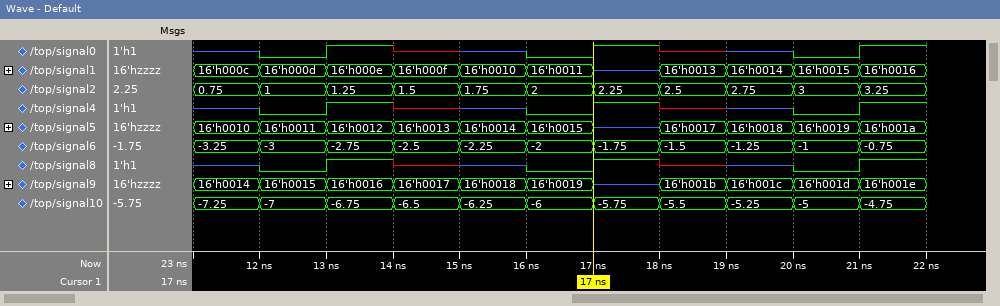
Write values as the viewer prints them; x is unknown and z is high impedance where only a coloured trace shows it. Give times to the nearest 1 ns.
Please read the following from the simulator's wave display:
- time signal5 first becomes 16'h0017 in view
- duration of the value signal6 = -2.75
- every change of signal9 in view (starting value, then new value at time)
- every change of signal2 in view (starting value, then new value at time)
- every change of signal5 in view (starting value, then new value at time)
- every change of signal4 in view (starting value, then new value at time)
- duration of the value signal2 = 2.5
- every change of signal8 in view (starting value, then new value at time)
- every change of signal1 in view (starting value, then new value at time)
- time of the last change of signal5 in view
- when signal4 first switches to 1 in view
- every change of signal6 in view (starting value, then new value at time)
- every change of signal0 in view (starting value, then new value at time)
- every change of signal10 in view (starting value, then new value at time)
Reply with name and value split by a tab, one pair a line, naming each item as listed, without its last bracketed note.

time signal5 first becomes 16'h0017 in view	18 ns
duration of the value signal6 = -2.75	1 ns
every change of signal9 in view	16'h0014, 16'h0015 at 12 ns, 16'h0016 at 13 ns, 16'h0017 at 14 ns, 16'h0018 at 15 ns, 16'h0019 at 16 ns, z at 17 ns, 16'h001b at 18 ns, 16'h001c at 19 ns, 16'h001d at 20 ns, 16'h001e at 21 ns
every change of signal2 in view	0.75, 1 at 12 ns, 1.25 at 13 ns, 1.5 at 14 ns, 1.75 at 15 ns, 2 at 16 ns, 2.25 at 17 ns, 2.5 at 18 ns, 2.75 at 19 ns, 3 at 20 ns, 3.25 at 21 ns
every change of signal5 in view	16'h0010, 16'h0011 at 12 ns, 16'h0012 at 13 ns, 16'h0013 at 14 ns, 16'h0014 at 15 ns, 16'h0015 at 16 ns, z at 17 ns, 16'h0017 at 18 ns, 16'h0018 at 19 ns, 16'h0019 at 20 ns, 16'h001a at 21 ns
every change of signal4 in view	z, 0 at 12 ns, 1 at 13 ns, x at 14 ns, z at 15 ns, 0 at 16 ns, 1 at 17 ns, x at 18 ns, z at 19 ns, 0 at 20 ns, 1 at 21 ns
duration of the value signal2 = 2.5	1 ns
every change of signal8 in view	z, 0 at 12 ns, 1 at 13 ns, x at 14 ns, z at 15 ns, 0 at 16 ns, 1 at 17 ns, x at 18 ns, z at 19 ns, 0 at 20 ns, 1 at 21 ns
every change of signal1 in view	16'h000c, 16'h000d at 12 ns, 16'h000e at 13 ns, 16'h000f at 14 ns, 16'h0010 at 15 ns, 16'h0011 at 16 ns, z at 17 ns, 16'h0013 at 18 ns, 16'h0014 at 19 ns, 16'h0015 at 20 ns, 16'h0016 at 21 ns
time of the last change of signal5 in view	21 ns
when signal4 first switches to 1 in view	13 ns
every change of signal6 in view	-3.25, -3 at 12 ns, -2.75 at 13 ns, -2.5 at 14 ns, -2.25 at 15 ns, -2 at 16 ns, -1.75 at 17 ns, -1.5 at 18 ns, -1.25 at 19 ns, -1 at 20 ns, -0.75 at 21 ns
every change of signal0 in view	z, 0 at 12 ns, 1 at 13 ns, x at 14 ns, z at 15 ns, 0 at 16 ns, 1 at 17 ns, x at 18 ns, z at 19 ns, 0 at 20 ns, 1 at 21 ns
every change of signal10 in view	-7.25, -7 at 12 ns, -6.75 at 13 ns, -6.5 at 14 ns, -6.25 at 15 ns, -6 at 16 ns, -5.75 at 17 ns, -5.5 at 18 ns, -5.25 at 19 ns, -5 at 20 ns, -4.75 at 21 ns
